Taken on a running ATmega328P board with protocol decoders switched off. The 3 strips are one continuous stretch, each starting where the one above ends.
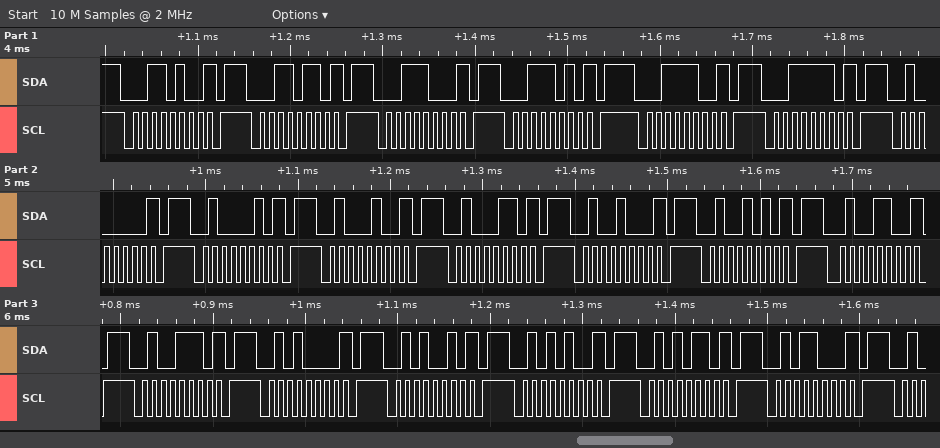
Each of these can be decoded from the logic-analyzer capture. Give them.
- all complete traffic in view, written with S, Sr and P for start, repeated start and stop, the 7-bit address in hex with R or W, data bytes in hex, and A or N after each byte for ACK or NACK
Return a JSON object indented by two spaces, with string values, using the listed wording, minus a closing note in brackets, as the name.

{
  "all complete traffic in view, written with S, Sr and P for start, repeated start and stop, the 7-bit address in hex with R or W, data bytes in hex, and A or N after each byte for ACK or NACK": "S 1AW N P S 1BW N P S 1CW N P S 1DW N P S 1EW N P S 1FW N P S 20W N P S 21W N P S 22W N P S 23W N P S 24W N P S 25W N P S 26W N P S 27W N P S 28W N P S 29W N P S 2AW N P S 2BW N P S 2CW N P"
}
